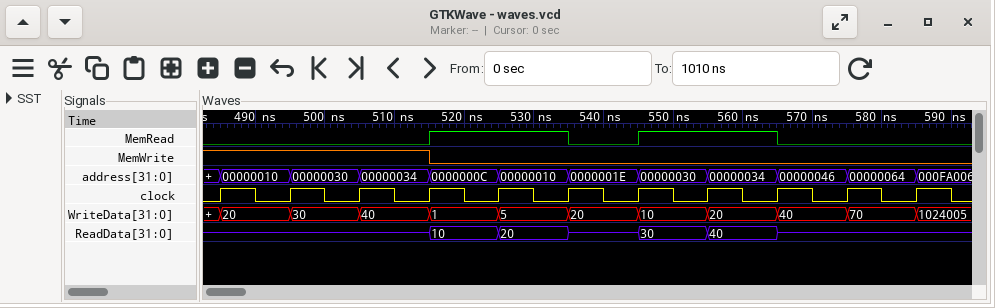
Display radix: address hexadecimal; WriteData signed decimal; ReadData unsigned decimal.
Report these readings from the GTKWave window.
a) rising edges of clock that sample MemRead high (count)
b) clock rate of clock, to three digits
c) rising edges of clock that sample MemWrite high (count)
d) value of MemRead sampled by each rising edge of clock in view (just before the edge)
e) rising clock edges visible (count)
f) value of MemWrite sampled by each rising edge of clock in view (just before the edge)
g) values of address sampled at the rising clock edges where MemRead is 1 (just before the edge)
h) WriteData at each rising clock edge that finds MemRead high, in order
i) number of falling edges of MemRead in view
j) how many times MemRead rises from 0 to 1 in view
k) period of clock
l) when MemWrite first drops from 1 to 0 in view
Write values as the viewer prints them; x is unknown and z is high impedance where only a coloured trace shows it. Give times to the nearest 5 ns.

4
100 MHz
4
0 0 0 0 1 1 0 1 1 0 0
11
1 1 1 1 0 0 0 0 0 0 0
0000000C, 00000010, 00000030, 00000034
1, 5, 10, 20
2
2
10 ns
515 ns
